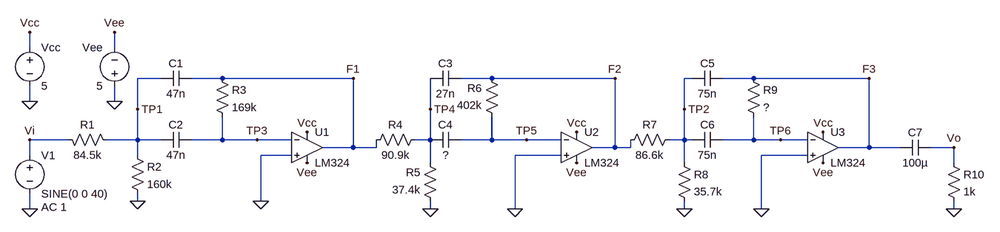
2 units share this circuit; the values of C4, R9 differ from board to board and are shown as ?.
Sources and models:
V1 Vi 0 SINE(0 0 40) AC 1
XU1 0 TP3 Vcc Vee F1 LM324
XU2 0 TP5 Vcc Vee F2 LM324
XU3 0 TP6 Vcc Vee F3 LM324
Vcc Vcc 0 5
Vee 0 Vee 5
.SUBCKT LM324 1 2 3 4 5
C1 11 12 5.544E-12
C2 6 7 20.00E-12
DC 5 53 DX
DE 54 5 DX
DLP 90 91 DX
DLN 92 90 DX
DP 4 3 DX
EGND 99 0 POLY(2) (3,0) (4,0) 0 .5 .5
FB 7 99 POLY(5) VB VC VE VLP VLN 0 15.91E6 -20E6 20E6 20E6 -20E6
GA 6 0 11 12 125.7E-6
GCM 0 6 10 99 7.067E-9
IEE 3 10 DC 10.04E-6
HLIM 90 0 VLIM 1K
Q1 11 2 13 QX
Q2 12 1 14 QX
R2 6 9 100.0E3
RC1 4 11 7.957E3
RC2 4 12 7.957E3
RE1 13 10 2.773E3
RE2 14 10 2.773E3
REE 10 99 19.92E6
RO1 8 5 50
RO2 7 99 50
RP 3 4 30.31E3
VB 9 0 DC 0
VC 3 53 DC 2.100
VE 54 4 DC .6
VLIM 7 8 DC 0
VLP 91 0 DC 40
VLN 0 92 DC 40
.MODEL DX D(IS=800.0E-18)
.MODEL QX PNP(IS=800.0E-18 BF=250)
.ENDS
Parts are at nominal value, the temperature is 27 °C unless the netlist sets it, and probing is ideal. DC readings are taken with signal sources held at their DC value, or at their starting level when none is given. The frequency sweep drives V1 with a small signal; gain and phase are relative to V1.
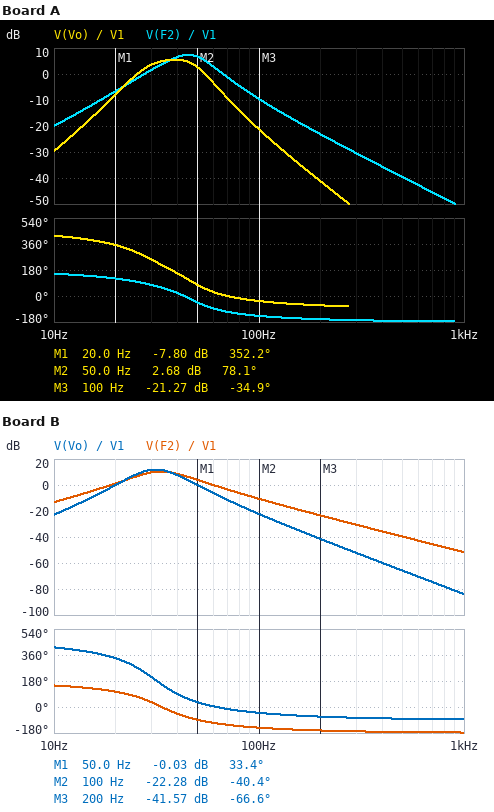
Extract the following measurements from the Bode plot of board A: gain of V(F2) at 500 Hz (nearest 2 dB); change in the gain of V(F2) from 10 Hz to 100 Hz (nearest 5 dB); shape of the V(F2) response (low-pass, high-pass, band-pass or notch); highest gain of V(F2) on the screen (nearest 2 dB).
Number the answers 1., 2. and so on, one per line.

1. -40 dB
2. 10 dB
3. band-pass
4. 8 dB
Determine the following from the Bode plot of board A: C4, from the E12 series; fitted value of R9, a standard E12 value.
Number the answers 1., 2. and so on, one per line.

1. 39 nF
2. 220 kΩ
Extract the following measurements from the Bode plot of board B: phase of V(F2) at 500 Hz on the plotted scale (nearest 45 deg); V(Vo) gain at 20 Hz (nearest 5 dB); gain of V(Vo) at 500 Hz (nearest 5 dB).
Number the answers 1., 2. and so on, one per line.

1. -180 deg
2. 0 dB
3. -65 dB
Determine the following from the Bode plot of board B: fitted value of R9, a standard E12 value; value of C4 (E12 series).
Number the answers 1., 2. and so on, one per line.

1. 220 kΩ
2. 82 nF
